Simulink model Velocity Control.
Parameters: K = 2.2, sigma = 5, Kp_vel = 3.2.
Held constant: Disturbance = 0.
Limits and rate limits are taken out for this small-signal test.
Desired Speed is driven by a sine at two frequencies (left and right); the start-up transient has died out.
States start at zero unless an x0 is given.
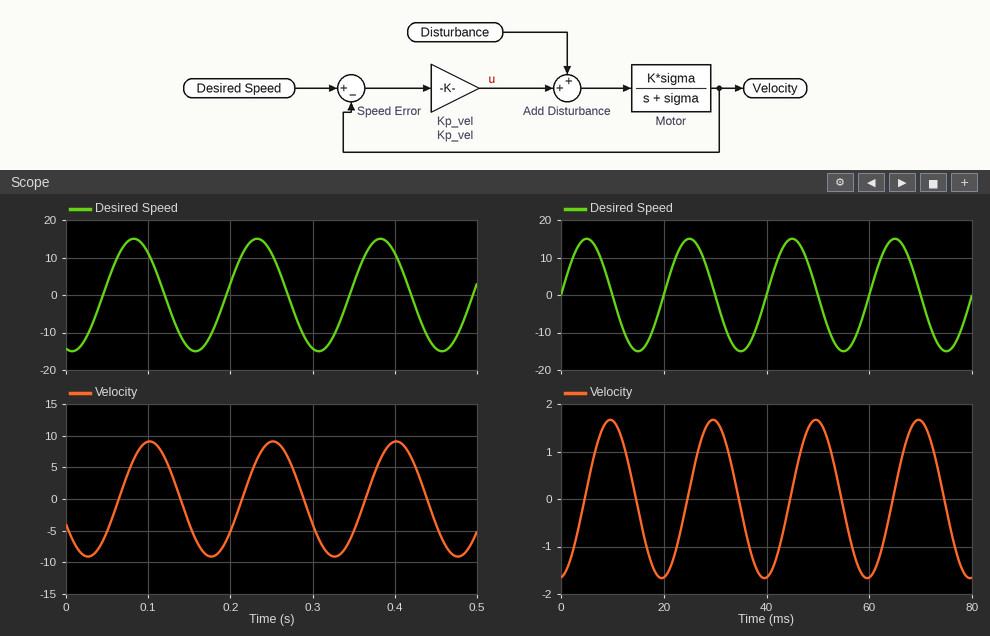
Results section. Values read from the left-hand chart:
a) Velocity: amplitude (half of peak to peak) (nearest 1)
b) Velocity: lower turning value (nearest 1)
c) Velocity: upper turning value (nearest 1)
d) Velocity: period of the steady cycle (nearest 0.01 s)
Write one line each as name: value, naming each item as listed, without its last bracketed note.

Velocity: amplitude (half of peak to peak): 9
Velocity: lower turning value: -9
Velocity: upper turning value: 9
Velocity: period of the steady cycle: 0.15 s
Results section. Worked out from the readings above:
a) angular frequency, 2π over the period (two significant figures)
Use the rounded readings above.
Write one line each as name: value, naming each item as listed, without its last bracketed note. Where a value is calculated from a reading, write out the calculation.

angular frequency, 2π over the period: 2π / 0.15 = 42 rad/s
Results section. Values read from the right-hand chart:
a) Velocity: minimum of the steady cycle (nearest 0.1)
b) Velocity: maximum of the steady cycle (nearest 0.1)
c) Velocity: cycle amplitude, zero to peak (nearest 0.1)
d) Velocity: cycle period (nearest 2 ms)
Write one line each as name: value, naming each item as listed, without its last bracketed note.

Velocity: minimum of the steady cycle: -1.7
Velocity: maximum of the steady cycle: 1.7
Velocity: cycle amplitude, zero to peak: 1.7
Velocity: cycle period: 20 ms
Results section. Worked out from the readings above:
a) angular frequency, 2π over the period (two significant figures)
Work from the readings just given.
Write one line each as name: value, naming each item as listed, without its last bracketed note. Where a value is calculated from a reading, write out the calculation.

angular frequency, 2π over the period: 2π / 20 = 0.31 rad/ms
